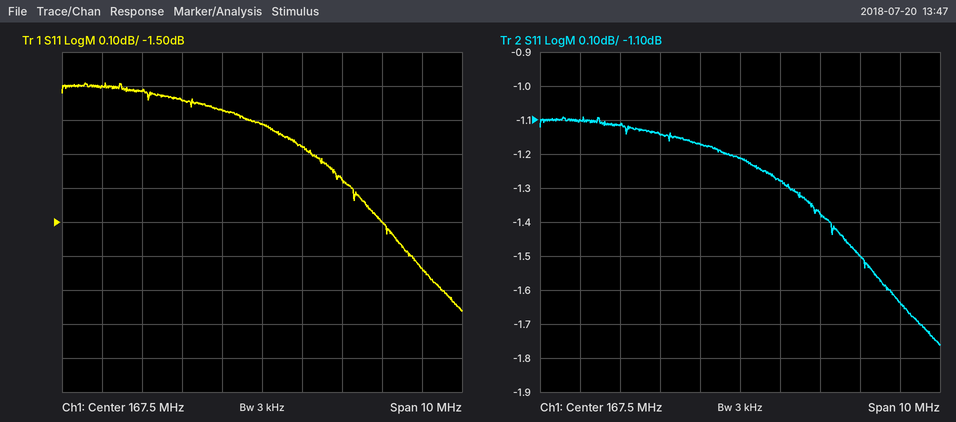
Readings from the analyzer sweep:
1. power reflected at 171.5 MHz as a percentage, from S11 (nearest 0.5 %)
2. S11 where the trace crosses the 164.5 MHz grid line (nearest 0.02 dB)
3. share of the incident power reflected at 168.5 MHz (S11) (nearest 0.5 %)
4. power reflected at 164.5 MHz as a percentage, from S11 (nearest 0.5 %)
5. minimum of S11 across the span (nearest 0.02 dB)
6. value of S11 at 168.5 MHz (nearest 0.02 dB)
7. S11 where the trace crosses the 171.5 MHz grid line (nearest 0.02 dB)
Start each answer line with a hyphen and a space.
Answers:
- 68.5 %
- -1.12 dB
- 74.5 %
- 77.5 %
- -1.76 dB
- -1.28 dB
- -1.64 dB
